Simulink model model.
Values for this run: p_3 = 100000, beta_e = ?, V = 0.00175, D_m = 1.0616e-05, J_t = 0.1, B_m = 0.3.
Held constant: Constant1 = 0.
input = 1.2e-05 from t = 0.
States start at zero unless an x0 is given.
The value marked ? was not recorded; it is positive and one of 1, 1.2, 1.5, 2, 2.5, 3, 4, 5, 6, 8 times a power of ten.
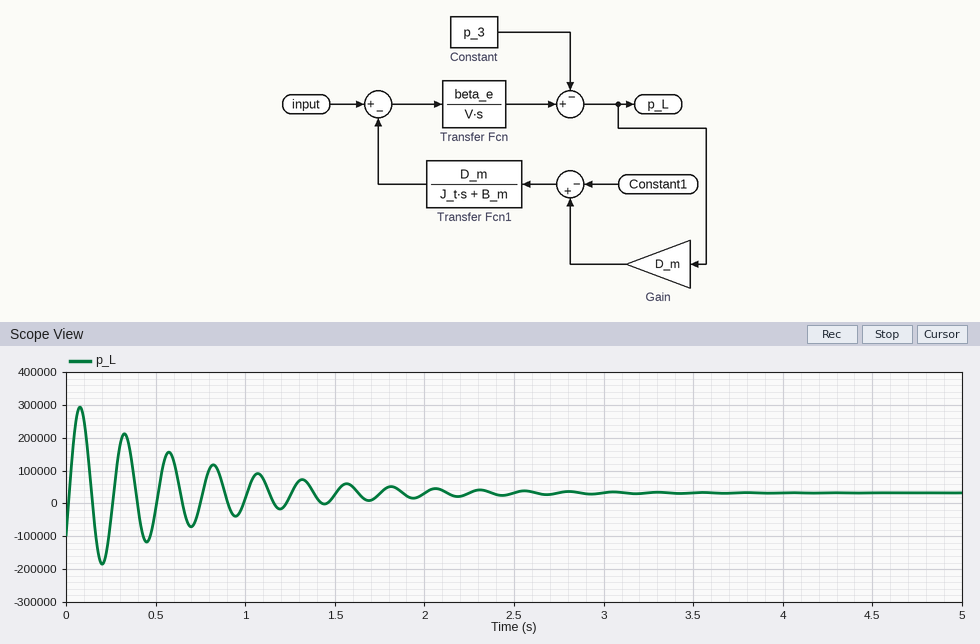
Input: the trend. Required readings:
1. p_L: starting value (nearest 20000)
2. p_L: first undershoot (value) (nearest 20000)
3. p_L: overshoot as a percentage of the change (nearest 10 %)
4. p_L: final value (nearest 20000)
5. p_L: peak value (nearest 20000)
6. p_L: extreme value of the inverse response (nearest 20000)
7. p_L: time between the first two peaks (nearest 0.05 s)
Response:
-100000
-180000
200 %
40000
300000
-180000
0.25 s
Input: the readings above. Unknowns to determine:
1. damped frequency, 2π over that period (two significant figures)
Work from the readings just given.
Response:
25 rad/s
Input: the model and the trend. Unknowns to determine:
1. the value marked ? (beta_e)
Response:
1e+09
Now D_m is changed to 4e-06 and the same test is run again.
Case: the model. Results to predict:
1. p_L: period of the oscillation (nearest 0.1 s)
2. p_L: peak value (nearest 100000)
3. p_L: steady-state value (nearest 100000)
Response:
0.7 s
800000
200000
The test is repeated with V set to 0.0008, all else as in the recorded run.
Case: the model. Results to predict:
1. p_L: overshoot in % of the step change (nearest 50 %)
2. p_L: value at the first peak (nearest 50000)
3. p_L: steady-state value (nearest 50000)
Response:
300 %
400000
50000
